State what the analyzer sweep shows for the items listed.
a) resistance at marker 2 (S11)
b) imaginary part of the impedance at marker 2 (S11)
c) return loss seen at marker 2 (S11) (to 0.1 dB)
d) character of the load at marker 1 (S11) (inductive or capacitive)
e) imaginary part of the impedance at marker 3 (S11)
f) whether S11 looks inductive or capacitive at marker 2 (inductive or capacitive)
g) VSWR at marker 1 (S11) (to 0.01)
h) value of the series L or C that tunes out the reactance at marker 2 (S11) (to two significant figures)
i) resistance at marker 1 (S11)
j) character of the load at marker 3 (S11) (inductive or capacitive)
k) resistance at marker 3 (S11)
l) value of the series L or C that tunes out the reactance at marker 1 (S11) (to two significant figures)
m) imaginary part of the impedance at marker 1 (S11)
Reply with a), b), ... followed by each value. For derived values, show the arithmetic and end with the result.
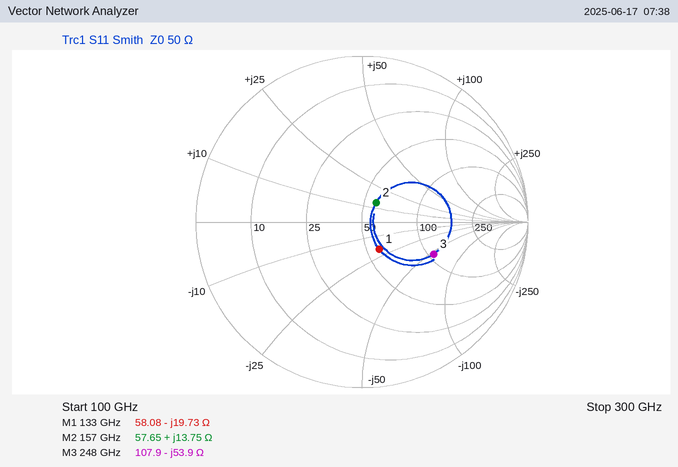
a) 57.65 Ω
b) +13.75 Ω
c) 16.8 dB
d) capacitive
e) -53.9 Ω
f) inductive
g) 1.48
h) C = 1/(2π × 157 GHz × 13.75 Ω) ≈ 74 fF
i) 58.08 Ω
j) capacitive
k) 107.9 Ω
l) L = 19.73 Ω/(2π × 133 GHz) ≈ 24 pH
m) -19.73 Ω
